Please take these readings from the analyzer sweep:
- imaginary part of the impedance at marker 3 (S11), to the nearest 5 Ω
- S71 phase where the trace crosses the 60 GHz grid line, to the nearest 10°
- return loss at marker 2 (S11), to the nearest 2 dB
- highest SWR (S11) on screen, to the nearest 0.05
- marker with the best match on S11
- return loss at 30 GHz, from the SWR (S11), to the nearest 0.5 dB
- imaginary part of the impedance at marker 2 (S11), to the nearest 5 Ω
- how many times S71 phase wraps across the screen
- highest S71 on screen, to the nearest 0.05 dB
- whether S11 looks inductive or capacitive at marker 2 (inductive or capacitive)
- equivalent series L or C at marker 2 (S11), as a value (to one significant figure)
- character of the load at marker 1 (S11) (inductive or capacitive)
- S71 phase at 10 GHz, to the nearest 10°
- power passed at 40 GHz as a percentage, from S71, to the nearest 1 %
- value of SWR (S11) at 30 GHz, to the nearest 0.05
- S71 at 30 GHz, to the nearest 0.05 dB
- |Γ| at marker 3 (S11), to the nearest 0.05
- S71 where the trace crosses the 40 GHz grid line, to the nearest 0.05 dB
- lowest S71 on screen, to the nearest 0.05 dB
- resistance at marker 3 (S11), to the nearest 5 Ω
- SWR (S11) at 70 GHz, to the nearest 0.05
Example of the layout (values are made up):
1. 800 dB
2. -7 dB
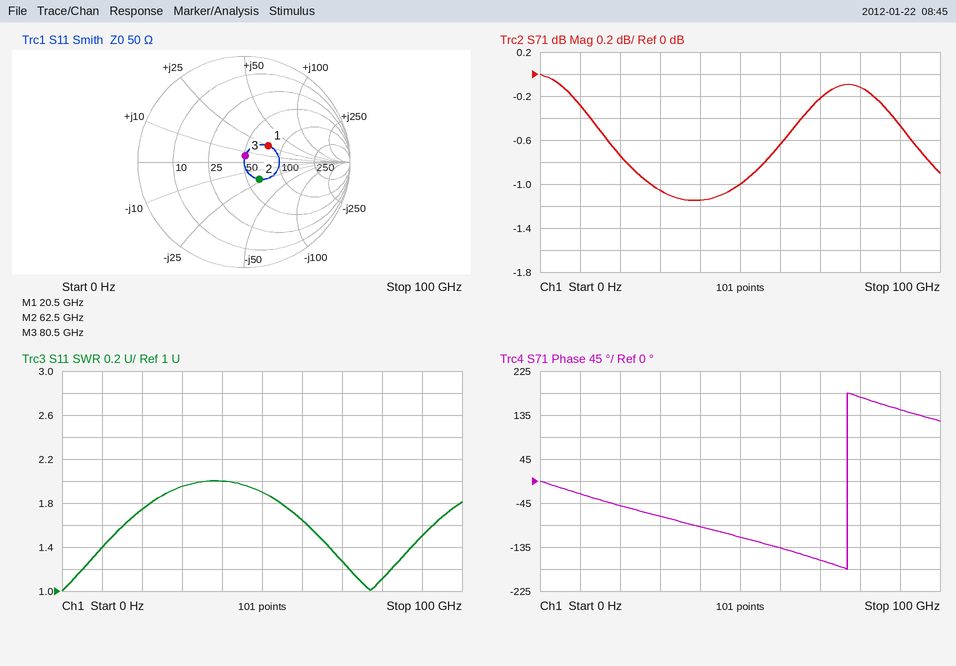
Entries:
1. +5 Ω
2. -140°
3. 14 dB
4. 2.00
5. marker 3
6. 10.0 dB
7. -20 Ω
8. 1
9. 0.00 dB
10. capacitive
11. 100 fF
12. inductive
13. -30°
14. 77 %
15. 1.95
16. -1.05 dB
17. 0.05
18. -1.15 dB
19. -1.15 dB
20. 50 Ω
21. 1.25
